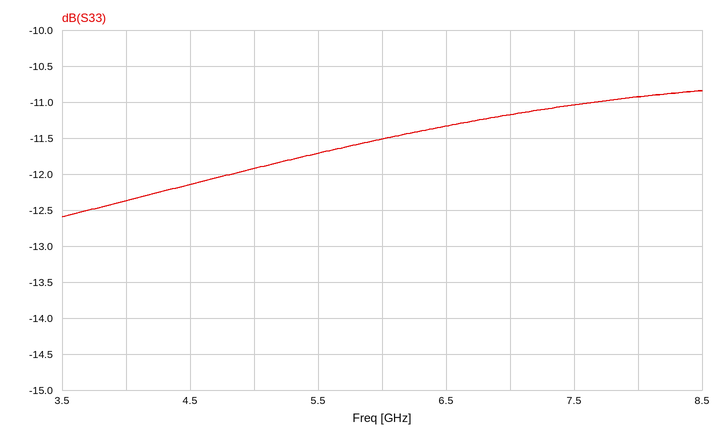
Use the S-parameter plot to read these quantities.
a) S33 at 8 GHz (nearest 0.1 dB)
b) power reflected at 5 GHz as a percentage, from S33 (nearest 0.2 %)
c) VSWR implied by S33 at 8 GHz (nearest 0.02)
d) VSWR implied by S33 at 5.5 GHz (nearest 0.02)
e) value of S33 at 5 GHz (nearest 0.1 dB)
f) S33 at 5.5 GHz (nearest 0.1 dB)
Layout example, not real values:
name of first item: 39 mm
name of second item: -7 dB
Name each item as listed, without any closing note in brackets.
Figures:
S33 at 8 GHz: -10.9 dB
power reflected at 5 GHz as a percentage, from S33: 6.4 %
VSWR implied by S33 at 8 GHz: 1.80
VSWR implied by S33 at 5.5 GHz: 1.70
value of S33 at 5 GHz: -11.9 dB
S33 at 5.5 GHz: -11.7 dB
